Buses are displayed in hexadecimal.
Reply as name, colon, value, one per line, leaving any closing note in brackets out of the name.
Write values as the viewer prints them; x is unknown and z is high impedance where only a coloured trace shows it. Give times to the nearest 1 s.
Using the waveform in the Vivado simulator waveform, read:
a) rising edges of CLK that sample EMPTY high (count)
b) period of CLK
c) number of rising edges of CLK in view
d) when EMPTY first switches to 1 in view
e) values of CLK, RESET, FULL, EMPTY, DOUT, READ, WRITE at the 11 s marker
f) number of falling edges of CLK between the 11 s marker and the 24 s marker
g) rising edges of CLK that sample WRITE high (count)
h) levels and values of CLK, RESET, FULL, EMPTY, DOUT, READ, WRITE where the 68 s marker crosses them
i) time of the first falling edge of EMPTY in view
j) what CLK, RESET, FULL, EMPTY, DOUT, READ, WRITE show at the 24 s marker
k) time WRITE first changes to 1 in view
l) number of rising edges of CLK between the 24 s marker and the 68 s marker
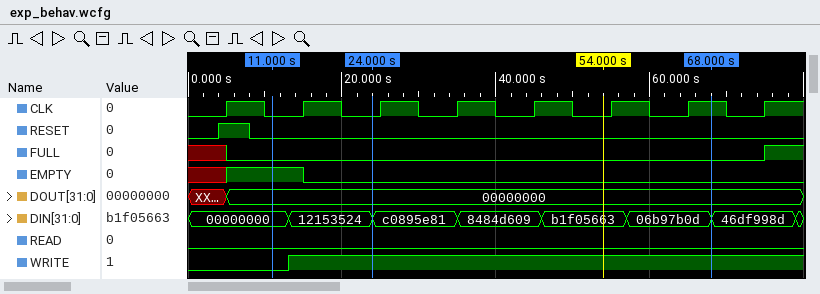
rising edges of CLK that sample EMPTY high: 1
period of CLK: 10 s
number of rising edges of CLK in view: 8
when EMPTY first switches to 1 in view: 5 s
values of CLK, RESET, FULL, EMPTY, DOUT, READ, WRITE at the 11 s marker: CLK=0, RESET=0, FULL=0, EMPTY=1, DOUT=00000000, READ=0, WRITE=0
number of falling edges of CLK between the 11 s marker and the 24 s marker: 1
rising edges of CLK that sample WRITE high: 7
levels and values of CLK, RESET, FULL, EMPTY, DOUT, READ, WRITE where the 68 s marker crosses them: CLK=1, RESET=0, FULL=0, EMPTY=0, DOUT=00000000, READ=0, WRITE=1
time of the first falling edge of EMPTY in view: 15 s
what CLK, RESET, FULL, EMPTY, DOUT, READ, WRITE show at the 24 s marker: CLK=0, RESET=0, FULL=0, EMPTY=0, DOUT=00000000, READ=0, WRITE=1
time WRITE first changes to 1 in view: 13 s
number of rising edges of CLK between the 24 s marker and the 68 s marker: 5
